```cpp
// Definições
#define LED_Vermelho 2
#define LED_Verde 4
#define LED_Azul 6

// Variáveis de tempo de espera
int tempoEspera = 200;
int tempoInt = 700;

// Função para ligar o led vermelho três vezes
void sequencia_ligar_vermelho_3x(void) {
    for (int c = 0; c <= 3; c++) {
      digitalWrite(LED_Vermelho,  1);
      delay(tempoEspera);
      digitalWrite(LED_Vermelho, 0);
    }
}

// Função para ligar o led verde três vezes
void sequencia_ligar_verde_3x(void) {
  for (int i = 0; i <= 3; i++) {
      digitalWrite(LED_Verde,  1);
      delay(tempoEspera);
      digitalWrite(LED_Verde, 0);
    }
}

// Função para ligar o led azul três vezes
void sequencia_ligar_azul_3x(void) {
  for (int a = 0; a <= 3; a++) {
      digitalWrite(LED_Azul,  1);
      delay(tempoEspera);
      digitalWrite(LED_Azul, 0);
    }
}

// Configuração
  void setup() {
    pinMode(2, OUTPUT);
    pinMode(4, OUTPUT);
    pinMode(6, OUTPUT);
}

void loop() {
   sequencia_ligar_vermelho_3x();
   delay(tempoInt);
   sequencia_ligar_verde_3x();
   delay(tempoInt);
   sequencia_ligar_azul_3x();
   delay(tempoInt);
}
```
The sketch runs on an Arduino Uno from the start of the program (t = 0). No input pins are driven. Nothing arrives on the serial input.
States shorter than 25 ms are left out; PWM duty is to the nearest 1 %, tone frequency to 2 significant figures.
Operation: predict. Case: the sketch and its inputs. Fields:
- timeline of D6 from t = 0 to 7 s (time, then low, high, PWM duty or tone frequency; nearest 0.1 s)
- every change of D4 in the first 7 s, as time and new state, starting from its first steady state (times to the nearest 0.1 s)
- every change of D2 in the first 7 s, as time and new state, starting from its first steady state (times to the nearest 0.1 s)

0 s low; 3 s high; 3.8 s low
0 s low; 1.5 s high; 2.3 s low; 6 s high; 6.8 s low
0 s high; 0.8 s low; 4.5 s high; 5.3 s low
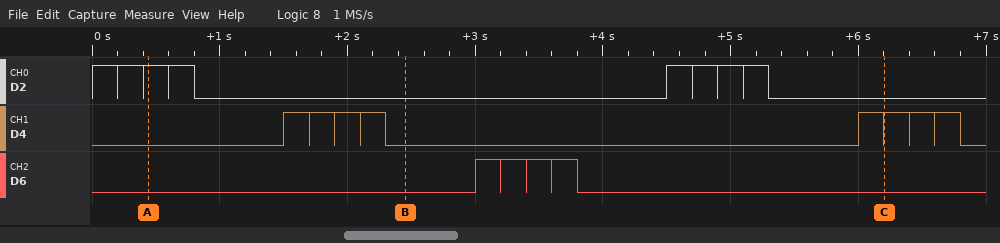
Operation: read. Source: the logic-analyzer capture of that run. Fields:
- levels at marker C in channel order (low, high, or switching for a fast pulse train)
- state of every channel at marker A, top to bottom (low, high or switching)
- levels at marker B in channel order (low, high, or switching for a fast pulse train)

D2 low, D4 high, D6 low
D2 high, D4 low, D6 low
D2 low, D4 low, D6 low
